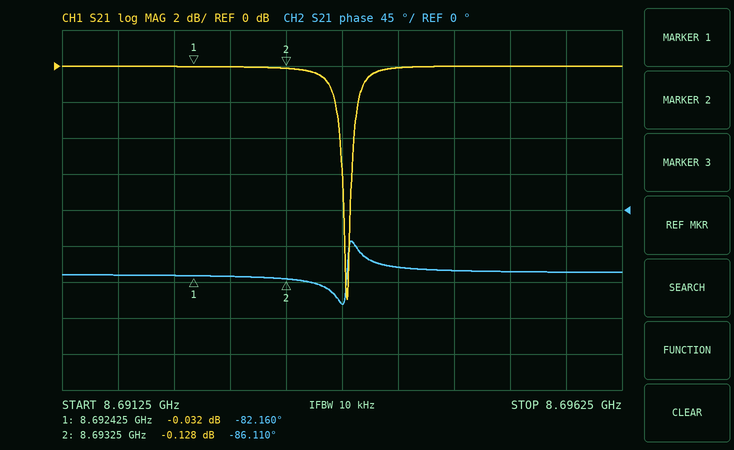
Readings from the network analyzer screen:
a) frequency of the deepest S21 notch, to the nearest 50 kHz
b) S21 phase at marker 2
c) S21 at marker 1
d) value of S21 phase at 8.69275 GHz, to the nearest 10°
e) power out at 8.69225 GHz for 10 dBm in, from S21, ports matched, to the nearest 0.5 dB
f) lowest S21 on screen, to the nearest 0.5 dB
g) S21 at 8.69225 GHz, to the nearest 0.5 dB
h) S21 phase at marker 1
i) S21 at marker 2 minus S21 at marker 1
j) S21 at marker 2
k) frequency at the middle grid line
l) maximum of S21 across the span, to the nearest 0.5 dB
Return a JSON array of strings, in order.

["8.69380 GHz", "-86.110°", "-0.032 dB", "-80°", "10.0 dBm", "-13.0 dB", "0.0 dB", "-82.160°", "-0.096 dB", "-0.128 dB", "8.69375 GHz", "0.0 dB"]
